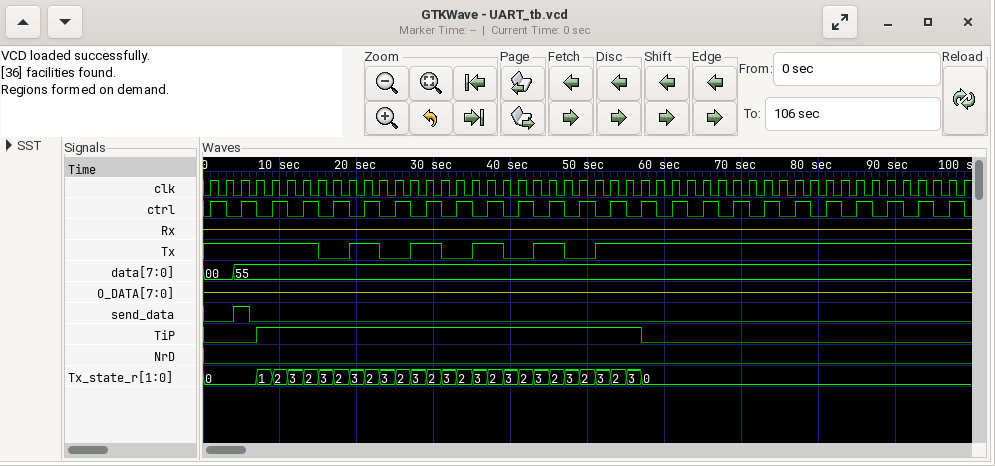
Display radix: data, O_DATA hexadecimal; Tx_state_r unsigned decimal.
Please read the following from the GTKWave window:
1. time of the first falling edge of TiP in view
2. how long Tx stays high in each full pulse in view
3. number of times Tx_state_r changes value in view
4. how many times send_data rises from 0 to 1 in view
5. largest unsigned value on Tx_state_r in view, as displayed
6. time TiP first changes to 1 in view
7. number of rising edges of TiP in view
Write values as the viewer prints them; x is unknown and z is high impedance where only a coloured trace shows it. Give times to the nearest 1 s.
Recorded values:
57 s
4 s, 4 s, 4 s, 4 s
26
1
3
7 s
1
